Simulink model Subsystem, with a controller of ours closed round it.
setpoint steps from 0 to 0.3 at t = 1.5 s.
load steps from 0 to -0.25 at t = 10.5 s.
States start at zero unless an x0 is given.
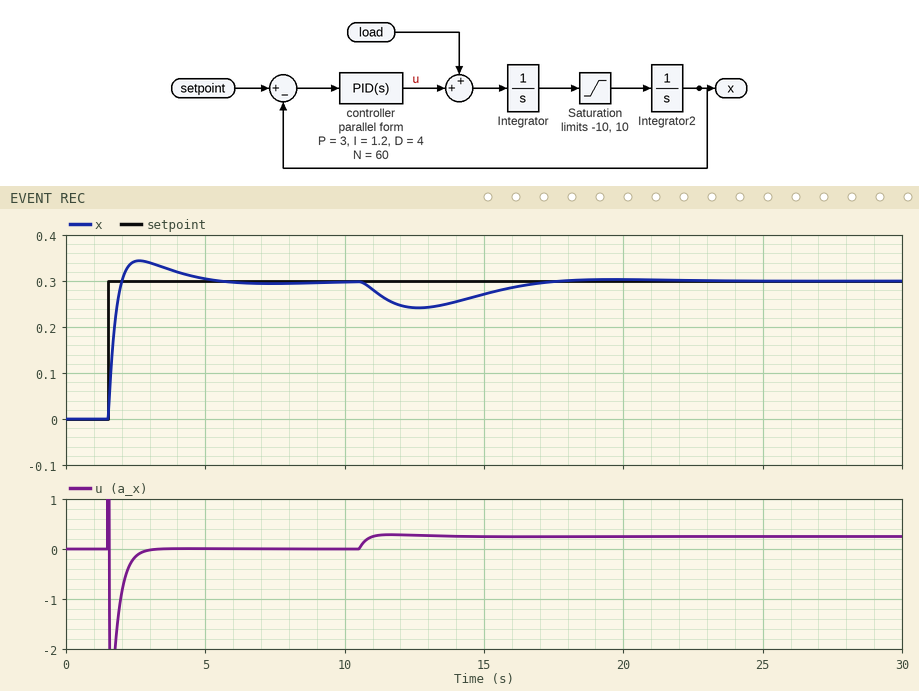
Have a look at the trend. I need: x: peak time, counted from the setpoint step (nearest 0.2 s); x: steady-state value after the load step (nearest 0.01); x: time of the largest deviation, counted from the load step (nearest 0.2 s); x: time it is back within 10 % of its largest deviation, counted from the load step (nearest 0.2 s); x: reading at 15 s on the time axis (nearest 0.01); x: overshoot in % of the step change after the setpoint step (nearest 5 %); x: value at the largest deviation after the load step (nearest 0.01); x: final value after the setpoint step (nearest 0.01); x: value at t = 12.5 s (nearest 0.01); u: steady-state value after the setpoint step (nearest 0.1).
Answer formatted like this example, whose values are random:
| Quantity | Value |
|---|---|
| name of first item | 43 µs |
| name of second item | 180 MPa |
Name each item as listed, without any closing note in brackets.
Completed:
| Quantity | Value |
|---|---|
| x: peak time, counted from the setpoint step | 1.2 s |
| x: steady-state value after the load step | 0.30 |
| x: time of the largest deviation, counted from the load step | 2.2 s |
| x: time it is back within 10 % of its largest deviation, counted from the load step | 6.4 s |
| x: reading at 15 s on the time axis | 0.27 |
| x: overshoot in % of the step change after the setpoint step | 15 % |
| x: value at the largest deviation after the load step | 0.24 |
| x: final value after the setpoint step | 0.30 |
| x: value at t = 12.5 s | 0.24 |
| u: steady-state value after the setpoint step | 0.0 |
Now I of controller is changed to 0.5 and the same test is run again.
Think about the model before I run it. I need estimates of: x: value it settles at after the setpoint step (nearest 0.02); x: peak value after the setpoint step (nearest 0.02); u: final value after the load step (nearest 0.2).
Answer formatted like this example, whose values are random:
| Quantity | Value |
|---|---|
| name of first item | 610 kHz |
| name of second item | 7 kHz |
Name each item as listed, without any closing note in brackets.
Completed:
| Quantity | Value |
|---|---|
| x: value it settles at after the setpoint step | 0.30 |
| x: peak value after the setpoint step | 0.34 |
| u: final value after the load step | 0.2 |
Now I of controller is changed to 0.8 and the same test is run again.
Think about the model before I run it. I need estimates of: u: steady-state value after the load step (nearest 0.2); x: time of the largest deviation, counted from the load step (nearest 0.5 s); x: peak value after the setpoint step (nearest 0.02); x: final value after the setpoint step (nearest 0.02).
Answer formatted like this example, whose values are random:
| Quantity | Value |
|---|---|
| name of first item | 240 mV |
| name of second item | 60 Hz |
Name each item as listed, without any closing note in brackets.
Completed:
| Quantity | Value |
|---|---|
| u: steady-state value after the load step | 0.2 |
| x: time of the largest deviation, counted from the load step | 2.5 s |
| x: peak value after the setpoint step | 0.34 |
| x: final value after the setpoint step | 0.30 |
